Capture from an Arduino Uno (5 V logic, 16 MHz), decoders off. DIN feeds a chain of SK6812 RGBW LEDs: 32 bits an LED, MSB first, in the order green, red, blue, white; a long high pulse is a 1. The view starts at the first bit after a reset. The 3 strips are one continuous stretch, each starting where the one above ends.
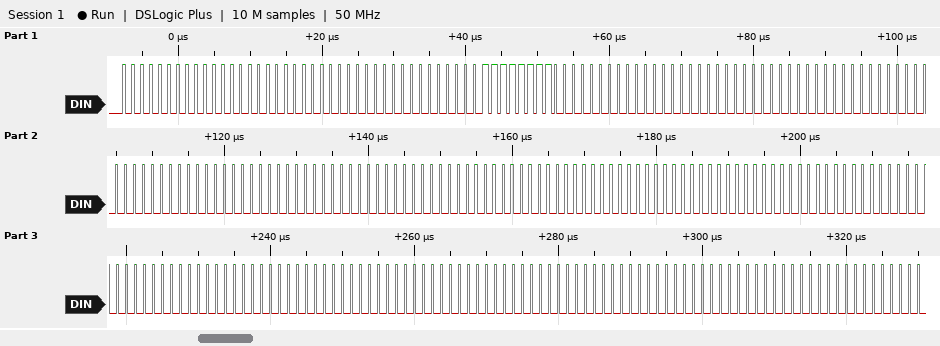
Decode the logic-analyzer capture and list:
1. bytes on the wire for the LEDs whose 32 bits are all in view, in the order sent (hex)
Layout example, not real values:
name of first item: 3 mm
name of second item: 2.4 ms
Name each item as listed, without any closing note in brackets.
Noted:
bytes on the wire for the LEDs whose 32 bits are all in view, in the order sent: 00 00 00 00 00 FF 00 00 00 00 00 00 00 00 00 00 00 00 00 00 00 00 00 00 00 00 00 00 00 00 00 00
